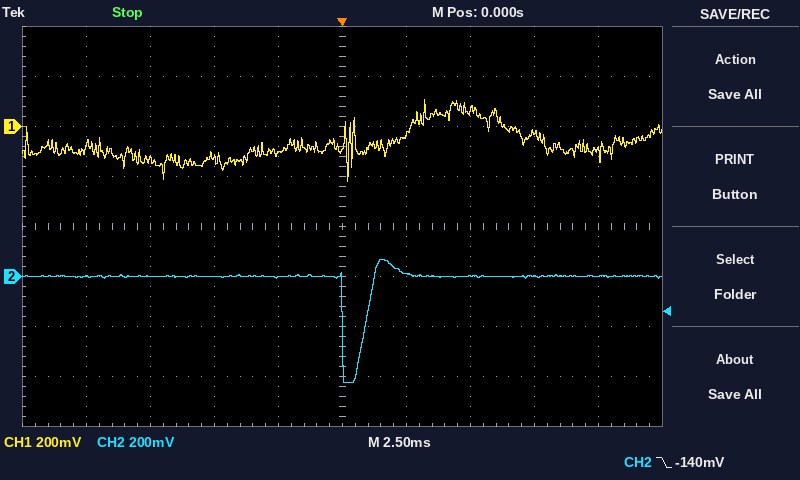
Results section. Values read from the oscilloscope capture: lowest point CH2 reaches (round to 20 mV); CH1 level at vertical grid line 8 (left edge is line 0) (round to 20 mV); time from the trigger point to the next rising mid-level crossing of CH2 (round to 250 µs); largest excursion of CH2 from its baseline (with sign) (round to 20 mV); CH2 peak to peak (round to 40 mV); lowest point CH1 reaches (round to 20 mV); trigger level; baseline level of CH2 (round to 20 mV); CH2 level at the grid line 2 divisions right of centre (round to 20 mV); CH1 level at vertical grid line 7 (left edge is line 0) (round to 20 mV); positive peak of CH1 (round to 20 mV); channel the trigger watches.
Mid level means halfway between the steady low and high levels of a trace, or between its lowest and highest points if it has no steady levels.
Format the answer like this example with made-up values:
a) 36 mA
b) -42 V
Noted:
a) -420 mV
b) -20 mV
c) 1.00 ms
d) -420 mV
e) 480 mV
f) -220 mV
g) -140 mV
h) 0 mV
i) 0 mV
j) 60 mV
k) 100 mV
l) CH2
